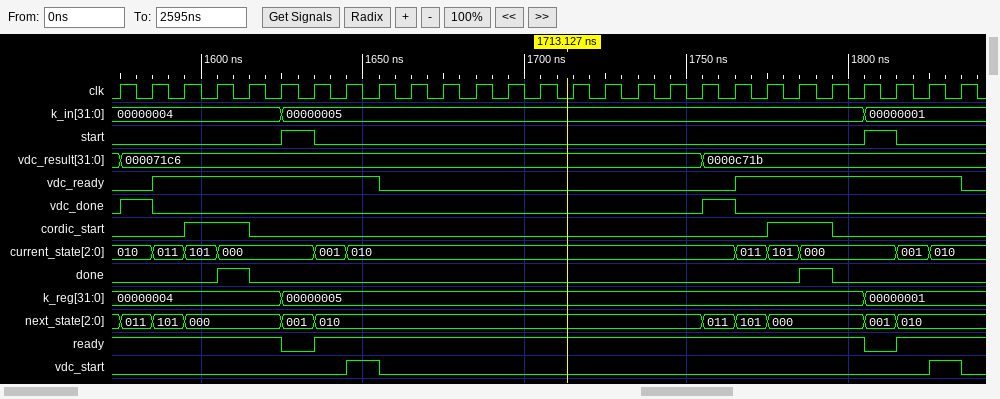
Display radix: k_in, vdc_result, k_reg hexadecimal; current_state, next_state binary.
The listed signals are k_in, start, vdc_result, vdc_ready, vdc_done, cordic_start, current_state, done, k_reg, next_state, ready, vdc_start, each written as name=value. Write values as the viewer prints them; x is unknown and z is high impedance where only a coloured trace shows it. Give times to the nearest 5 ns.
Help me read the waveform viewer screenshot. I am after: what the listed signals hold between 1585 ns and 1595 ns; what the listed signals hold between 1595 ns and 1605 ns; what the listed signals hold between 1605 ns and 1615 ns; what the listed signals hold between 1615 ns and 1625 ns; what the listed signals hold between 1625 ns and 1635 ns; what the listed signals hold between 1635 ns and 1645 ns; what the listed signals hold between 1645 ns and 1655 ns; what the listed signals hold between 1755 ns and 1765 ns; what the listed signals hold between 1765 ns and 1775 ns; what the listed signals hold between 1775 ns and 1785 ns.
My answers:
k_in=00000004, start=0, vdc_result=000071c6, vdc_ready=1, vdc_done=0, cordic_start=0, current_state=011, done=0, k_reg=00000004, next_state=101, ready=1, vdc_start=0
k_in=00000004, start=0, vdc_result=000071c6, vdc_ready=1, vdc_done=0, cordic_start=1, current_state=101, done=0, k_reg=00000004, next_state=000, ready=1, vdc_start=0
k_in=00000004, start=0, vdc_result=000071c6, vdc_ready=1, vdc_done=0, cordic_start=1, current_state=000, done=1, k_reg=00000004, next_state=000, ready=1, vdc_start=0
k_in=00000004, start=0, vdc_result=000071c6, vdc_ready=1, vdc_done=0, cordic_start=0, current_state=000, done=0, k_reg=00000004, next_state=000, ready=1, vdc_start=0
k_in=00000005, start=1, vdc_result=000071c6, vdc_ready=1, vdc_done=0, cordic_start=0, current_state=000, done=0, k_reg=00000005, next_state=001, ready=0, vdc_start=0
k_in=00000005, start=0, vdc_result=000071c6, vdc_ready=1, vdc_done=0, cordic_start=0, current_state=001, done=0, k_reg=00000005, next_state=010, ready=1, vdc_start=0
k_in=00000005, start=0, vdc_result=000071c6, vdc_ready=1, vdc_done=0, cordic_start=0, current_state=010, done=0, k_reg=00000005, next_state=010, ready=1, vdc_start=1
k_in=00000005, start=0, vdc_result=0000c71b, vdc_ready=0, vdc_done=1, cordic_start=0, current_state=010, done=0, k_reg=00000005, next_state=011, ready=1, vdc_start=0
k_in=00000005, start=0, vdc_result=0000c71b, vdc_ready=1, vdc_done=0, cordic_start=0, current_state=011, done=0, k_reg=00000005, next_state=101, ready=1, vdc_start=0
k_in=00000005, start=0, vdc_result=0000c71b, vdc_ready=1, vdc_done=0, cordic_start=1, current_state=101, done=0, k_reg=00000005, next_state=000, ready=1, vdc_start=0
